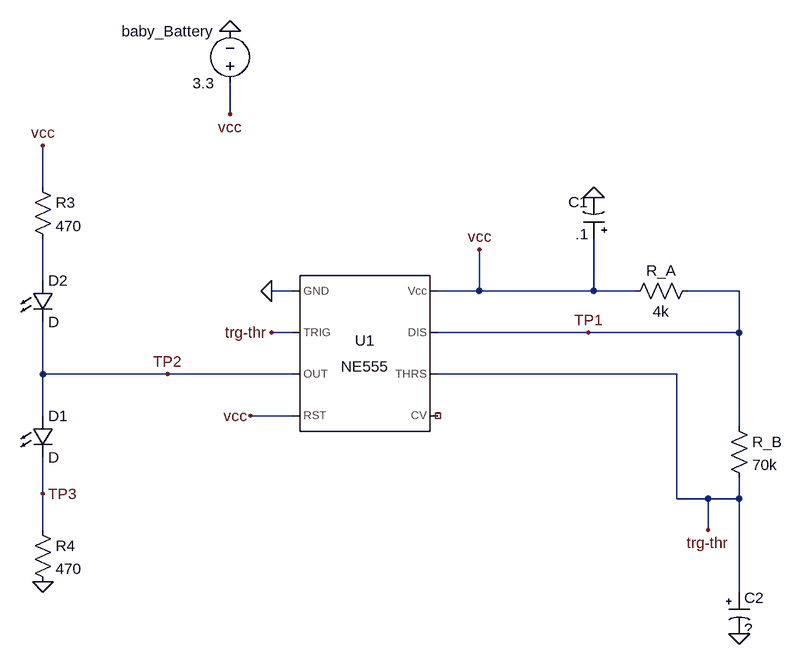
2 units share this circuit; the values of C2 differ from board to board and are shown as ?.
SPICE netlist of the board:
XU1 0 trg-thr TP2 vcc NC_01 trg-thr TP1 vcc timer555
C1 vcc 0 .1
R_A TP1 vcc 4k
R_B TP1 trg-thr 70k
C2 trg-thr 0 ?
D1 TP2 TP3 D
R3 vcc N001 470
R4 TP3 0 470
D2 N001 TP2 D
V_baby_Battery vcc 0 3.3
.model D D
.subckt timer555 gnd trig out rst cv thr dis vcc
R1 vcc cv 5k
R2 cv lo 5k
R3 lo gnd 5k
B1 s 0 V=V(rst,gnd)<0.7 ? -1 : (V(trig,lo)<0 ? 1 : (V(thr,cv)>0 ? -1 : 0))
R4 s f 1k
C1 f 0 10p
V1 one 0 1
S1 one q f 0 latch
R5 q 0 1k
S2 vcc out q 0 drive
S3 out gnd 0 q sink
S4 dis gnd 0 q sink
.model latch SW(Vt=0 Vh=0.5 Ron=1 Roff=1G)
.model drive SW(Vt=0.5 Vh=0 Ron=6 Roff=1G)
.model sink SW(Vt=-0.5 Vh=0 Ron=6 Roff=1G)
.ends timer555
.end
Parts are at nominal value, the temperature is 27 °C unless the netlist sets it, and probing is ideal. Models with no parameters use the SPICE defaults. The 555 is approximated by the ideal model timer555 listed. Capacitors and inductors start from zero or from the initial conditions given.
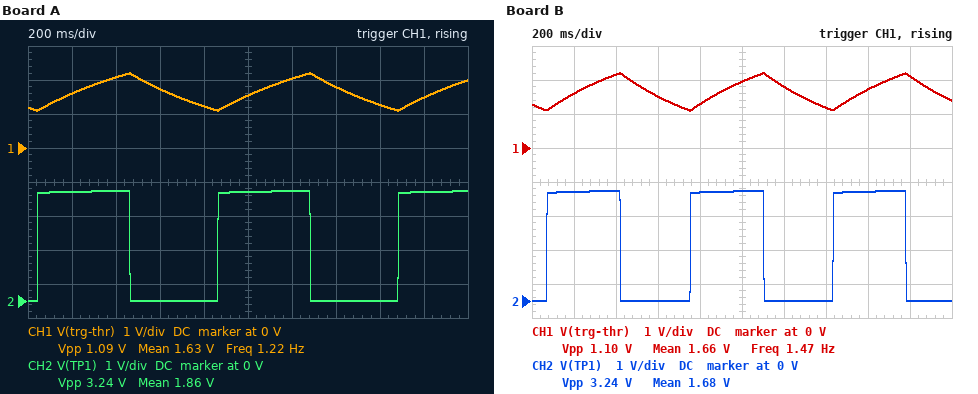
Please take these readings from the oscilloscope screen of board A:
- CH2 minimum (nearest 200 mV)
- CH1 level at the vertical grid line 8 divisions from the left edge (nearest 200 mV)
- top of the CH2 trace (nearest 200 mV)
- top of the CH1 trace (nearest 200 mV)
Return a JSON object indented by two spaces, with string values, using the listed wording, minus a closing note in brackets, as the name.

{
  "CH2 minimum": "0 V",
  "CH1 level at the vertical grid line 8 divisions from the left edge": "1.2 V",
  "top of the CH2 trace": "3.2 V",
  "top of the CH1 trace": "2.2 V"
}
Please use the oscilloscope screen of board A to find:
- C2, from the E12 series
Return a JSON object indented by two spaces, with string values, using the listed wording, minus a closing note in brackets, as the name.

{
  "C2, from the E12 series": "8.2 µF"
}
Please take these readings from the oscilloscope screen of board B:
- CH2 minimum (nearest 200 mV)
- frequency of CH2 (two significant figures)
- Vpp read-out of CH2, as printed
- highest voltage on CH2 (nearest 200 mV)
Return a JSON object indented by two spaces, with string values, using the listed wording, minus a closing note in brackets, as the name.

{
  "CH2 minimum": "0 V",
  "frequency of CH2": "1.5 Hz",
  "Vpp read-out of CH2, as printed": "3.24 V",
  "highest voltage on CH2": "3.2 V"
}
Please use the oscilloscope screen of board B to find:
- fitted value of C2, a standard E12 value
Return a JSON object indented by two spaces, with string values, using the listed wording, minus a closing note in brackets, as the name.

{
  "fitted value of C2, a standard E12 value": "6.8 µF"
}
